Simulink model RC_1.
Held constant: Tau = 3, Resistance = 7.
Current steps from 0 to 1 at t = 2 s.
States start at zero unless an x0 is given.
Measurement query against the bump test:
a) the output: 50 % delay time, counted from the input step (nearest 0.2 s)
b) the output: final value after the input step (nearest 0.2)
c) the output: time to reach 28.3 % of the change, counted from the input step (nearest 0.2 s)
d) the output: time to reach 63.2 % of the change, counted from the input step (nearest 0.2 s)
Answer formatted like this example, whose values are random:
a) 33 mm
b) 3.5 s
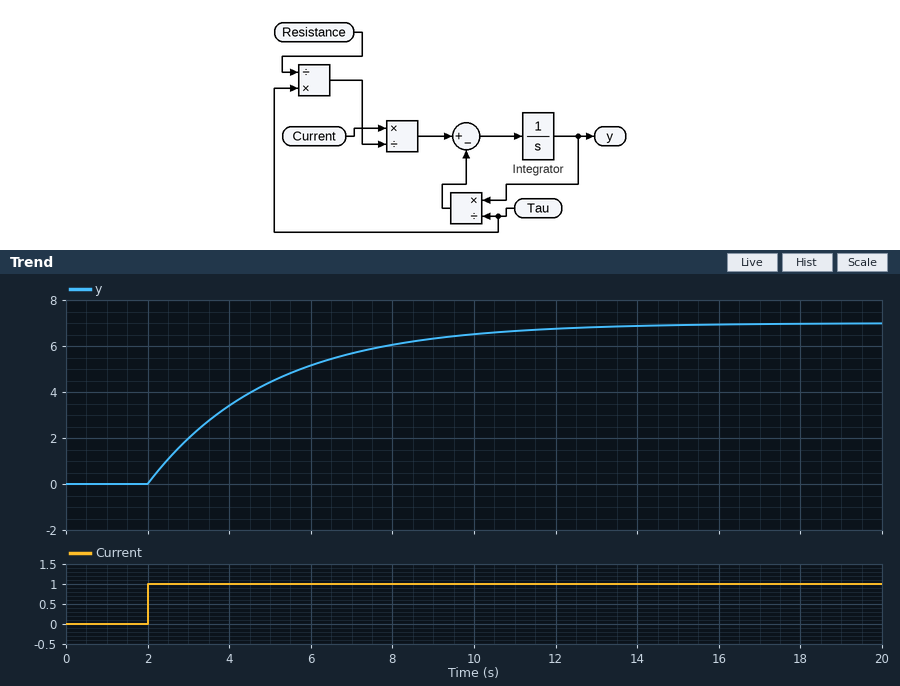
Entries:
a) 2.0 s
b) 7.0
c) 1.0 s
d) 3.0 s
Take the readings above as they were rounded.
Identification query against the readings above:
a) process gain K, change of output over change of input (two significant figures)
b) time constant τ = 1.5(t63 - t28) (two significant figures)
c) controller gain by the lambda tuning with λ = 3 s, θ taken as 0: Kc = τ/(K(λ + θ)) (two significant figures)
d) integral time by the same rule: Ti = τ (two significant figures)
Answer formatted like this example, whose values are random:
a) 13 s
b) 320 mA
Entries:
a) 7.0
b) 3.0 s
c) 0.14
d) 3.0 s
